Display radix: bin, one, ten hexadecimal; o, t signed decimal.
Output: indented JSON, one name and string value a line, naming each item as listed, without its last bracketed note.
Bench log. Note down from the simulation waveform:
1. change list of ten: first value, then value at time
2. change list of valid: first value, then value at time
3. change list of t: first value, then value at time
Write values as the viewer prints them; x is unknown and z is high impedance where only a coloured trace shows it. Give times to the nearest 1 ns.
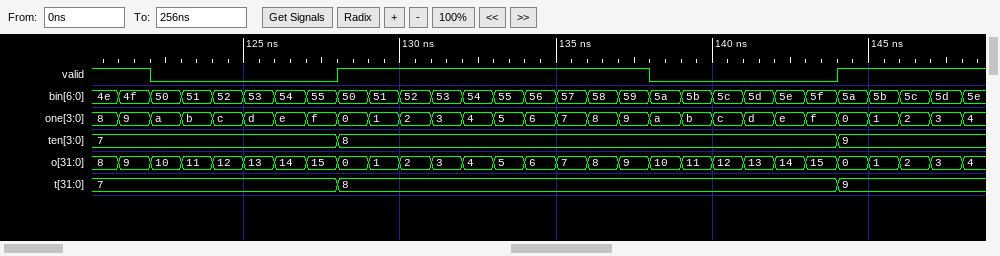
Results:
{
  "change list of ten: first value, then value at time": "7, 8 at 128 ns, 9 at 144 ns",
  "change list of valid: first value, then value at time": "1, 0 at 122 ns, 1 at 128 ns, 0 at 138 ns, 1 at 144 ns",
  "change list of t: first value, then value at time": "7, 8 at 128 ns, 9 at 144 ns"
}
